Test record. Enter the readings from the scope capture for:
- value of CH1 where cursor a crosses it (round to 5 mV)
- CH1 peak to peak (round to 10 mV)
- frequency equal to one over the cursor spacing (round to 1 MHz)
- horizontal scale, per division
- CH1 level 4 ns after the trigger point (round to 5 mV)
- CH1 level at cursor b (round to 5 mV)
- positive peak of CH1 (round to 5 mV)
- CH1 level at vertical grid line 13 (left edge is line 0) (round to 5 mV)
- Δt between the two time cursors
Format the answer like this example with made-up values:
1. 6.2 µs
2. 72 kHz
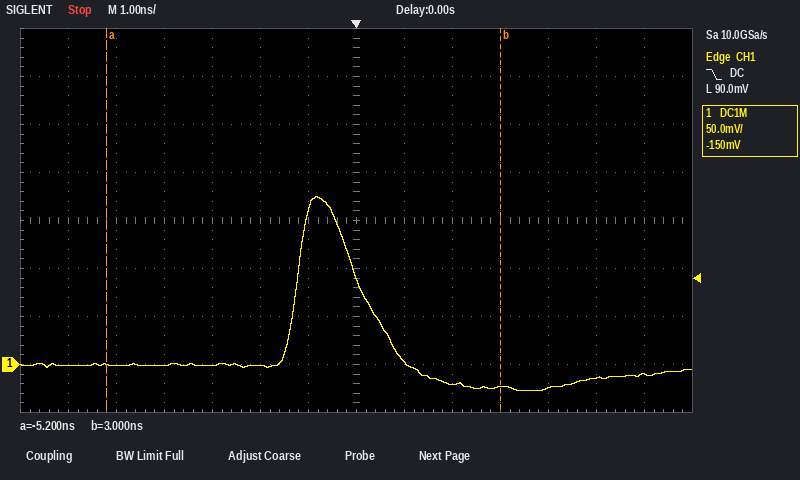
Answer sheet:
1. 0 mV
2. 200 mV
3. 122 MHz
4. 1 ns
5. -25 mV
6. -25 mV
7. 175 mV
8. -10 mV
9. 8.2 ns
